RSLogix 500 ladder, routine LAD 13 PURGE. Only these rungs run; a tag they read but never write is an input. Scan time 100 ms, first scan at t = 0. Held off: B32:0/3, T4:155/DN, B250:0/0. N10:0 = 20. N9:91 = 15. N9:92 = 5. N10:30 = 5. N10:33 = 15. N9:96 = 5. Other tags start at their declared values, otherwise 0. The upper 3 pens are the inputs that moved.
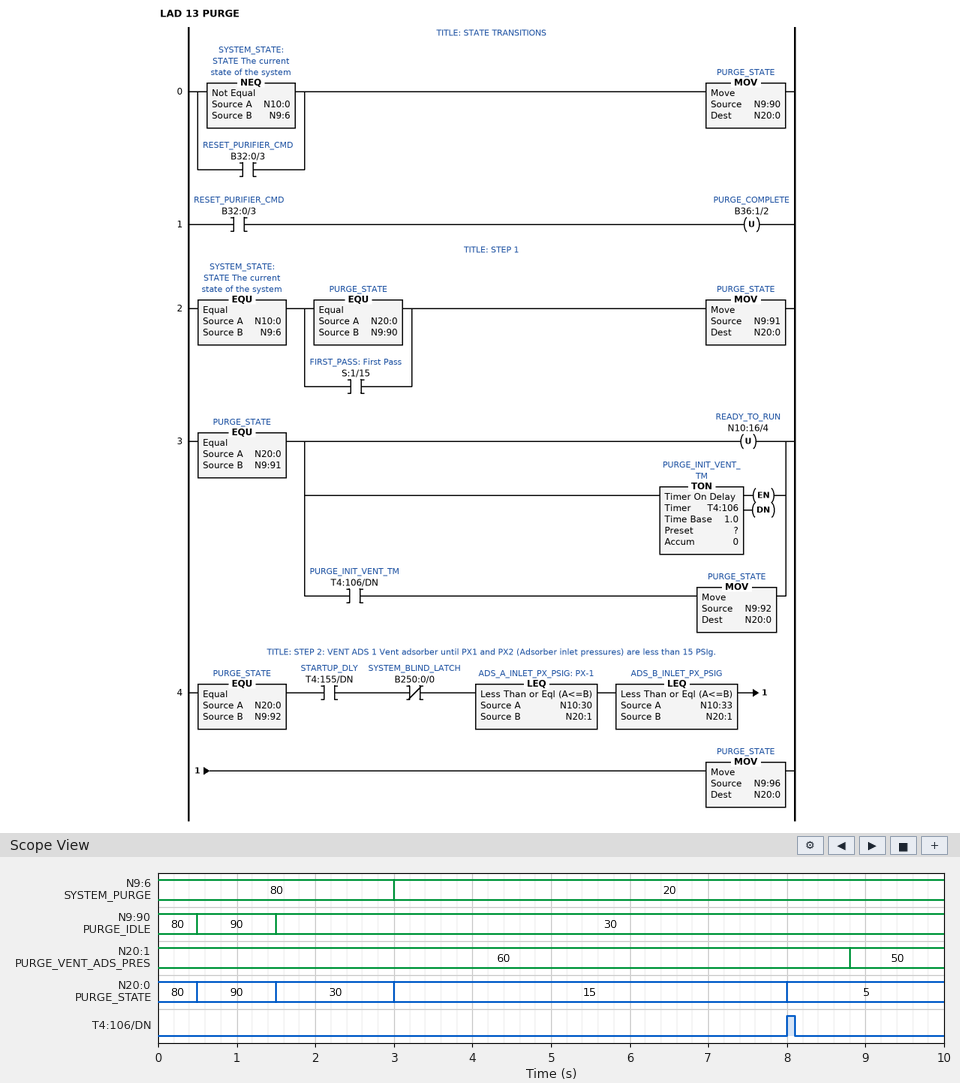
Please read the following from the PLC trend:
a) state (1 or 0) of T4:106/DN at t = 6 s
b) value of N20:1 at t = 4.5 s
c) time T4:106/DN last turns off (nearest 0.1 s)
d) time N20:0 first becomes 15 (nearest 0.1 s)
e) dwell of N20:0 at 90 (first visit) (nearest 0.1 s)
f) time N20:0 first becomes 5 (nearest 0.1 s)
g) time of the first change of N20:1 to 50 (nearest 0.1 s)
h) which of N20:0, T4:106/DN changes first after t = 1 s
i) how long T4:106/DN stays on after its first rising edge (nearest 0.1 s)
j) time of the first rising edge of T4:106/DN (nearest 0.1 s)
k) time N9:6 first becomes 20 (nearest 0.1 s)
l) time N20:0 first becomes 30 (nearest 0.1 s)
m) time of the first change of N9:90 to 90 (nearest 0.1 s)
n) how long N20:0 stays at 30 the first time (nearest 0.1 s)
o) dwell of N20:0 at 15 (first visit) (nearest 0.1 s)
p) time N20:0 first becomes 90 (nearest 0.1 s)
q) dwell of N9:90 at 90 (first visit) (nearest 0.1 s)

0
60
8.1 s
3.0 s
1.0 s
8.0 s
8.8 s
N20:0
0.1 s
8.0 s
3.0 s
1.5 s
0.5 s
1.5 s
5.0 s
0.5 s
1.0 s
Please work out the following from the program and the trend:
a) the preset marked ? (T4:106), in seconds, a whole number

5 s
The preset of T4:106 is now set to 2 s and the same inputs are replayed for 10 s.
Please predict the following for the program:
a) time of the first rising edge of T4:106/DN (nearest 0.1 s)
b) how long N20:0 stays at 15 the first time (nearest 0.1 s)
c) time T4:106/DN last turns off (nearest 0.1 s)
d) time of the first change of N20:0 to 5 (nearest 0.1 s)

5.0 s
2.0 s
5.1 s
5.0 s
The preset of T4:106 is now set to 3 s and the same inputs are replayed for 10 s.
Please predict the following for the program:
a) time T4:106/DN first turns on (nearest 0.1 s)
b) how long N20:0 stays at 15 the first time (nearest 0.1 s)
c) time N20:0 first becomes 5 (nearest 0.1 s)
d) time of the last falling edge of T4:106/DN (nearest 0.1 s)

6.0 s
3.0 s
6.0 s
6.1 s
